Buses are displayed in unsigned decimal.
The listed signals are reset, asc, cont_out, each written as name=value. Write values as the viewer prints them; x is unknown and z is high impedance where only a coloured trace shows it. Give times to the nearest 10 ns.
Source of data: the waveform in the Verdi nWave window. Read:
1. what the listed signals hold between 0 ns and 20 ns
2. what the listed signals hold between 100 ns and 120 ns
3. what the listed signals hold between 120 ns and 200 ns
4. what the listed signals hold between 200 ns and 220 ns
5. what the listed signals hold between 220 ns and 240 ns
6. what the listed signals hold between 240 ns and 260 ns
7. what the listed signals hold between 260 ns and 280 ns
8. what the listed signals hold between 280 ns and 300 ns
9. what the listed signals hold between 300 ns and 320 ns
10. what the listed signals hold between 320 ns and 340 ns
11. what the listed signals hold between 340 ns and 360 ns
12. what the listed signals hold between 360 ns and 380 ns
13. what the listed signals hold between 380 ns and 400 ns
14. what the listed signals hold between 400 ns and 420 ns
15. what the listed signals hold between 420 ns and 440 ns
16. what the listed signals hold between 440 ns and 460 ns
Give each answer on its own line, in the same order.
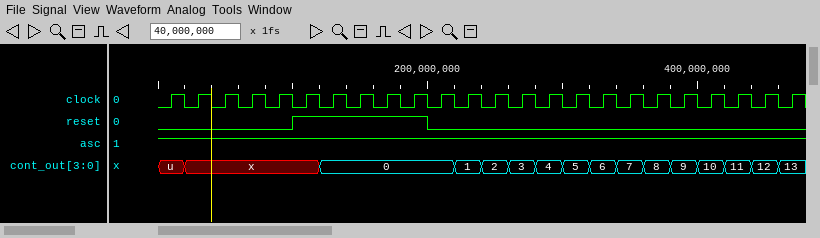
reset=0, asc=1, cont_out=u
reset=1, asc=1, cont_out=x
reset=1, asc=1, cont_out=0
reset=0, asc=1, cont_out=0
reset=0, asc=1, cont_out=1
reset=0, asc=1, cont_out=2
reset=0, asc=1, cont_out=3
reset=0, asc=1, cont_out=4
reset=0, asc=1, cont_out=5
reset=0, asc=1, cont_out=6
reset=0, asc=1, cont_out=7
reset=0, asc=1, cont_out=8
reset=0, asc=1, cont_out=9
reset=0, asc=1, cont_out=10
reset=0, asc=1, cont_out=11
reset=0, asc=1, cont_out=12
